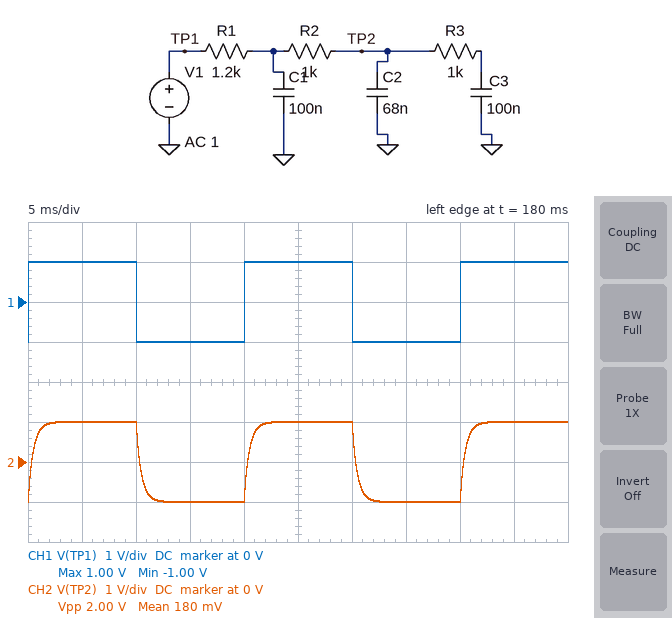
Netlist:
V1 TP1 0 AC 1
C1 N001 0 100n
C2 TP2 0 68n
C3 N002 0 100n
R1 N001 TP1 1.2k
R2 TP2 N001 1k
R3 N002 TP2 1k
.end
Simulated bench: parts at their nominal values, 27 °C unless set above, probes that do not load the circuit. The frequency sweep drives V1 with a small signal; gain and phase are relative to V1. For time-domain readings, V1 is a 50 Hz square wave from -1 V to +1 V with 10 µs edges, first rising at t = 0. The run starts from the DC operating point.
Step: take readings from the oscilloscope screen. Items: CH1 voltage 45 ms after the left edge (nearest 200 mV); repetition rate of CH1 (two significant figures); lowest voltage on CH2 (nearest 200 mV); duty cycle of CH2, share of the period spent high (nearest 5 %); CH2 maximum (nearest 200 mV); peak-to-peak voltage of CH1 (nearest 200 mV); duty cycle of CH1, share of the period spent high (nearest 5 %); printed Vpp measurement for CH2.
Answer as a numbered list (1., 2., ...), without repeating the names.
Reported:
1. 1.0 V
2. 50 Hz
3. -1.0 V
4. 50 %
5. 1.0 V
6. 2.0 V
7. 50 %
8. 2.00 V
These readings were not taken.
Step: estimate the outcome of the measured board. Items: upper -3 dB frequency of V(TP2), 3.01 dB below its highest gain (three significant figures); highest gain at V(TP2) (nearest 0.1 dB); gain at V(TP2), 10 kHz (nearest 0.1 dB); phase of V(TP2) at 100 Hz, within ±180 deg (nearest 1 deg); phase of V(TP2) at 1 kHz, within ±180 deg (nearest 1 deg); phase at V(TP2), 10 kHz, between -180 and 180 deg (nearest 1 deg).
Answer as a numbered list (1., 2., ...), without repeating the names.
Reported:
1. 326 Hz
2. 0 dB
3. -31.8 dB
4. -17 deg
5. -72 deg
6. -141 deg
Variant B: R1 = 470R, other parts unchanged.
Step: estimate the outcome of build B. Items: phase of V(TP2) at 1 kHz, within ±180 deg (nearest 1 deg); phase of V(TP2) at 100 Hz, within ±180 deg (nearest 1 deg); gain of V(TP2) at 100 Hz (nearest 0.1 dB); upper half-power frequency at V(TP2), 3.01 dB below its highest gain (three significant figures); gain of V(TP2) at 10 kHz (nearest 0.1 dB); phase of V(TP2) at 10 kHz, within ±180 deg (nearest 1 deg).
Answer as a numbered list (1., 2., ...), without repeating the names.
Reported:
1. -55 deg
2. -10 deg
3. -0.2 dB
4. 522 Hz
5. -24.2 dB
6. -131 deg
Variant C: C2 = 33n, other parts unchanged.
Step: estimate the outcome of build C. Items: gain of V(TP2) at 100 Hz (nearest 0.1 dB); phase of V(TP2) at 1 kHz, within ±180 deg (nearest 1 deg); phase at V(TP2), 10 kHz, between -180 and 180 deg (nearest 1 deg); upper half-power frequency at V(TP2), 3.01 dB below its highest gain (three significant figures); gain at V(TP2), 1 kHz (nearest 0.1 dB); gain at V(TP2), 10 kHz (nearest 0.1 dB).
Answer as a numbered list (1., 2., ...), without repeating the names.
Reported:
1. -0.3 dB
2. -65 deg
3. -125 deg
4. 378 Hz
5. -8.5 dB
6. -27.6 dB
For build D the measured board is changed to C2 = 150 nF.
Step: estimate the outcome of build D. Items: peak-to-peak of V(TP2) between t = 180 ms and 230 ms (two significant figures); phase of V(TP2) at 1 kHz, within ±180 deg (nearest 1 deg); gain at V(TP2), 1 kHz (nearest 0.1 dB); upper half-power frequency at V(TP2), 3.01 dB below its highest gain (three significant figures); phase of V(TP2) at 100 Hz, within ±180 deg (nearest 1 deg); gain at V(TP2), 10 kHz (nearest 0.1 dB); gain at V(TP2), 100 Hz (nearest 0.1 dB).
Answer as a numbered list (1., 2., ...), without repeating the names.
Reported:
1. 2.0 V
2. -82 deg
3. -12.2 dB
4. 243 Hz
5. -23 deg
6. -37.8 dB
7. -0.7 dB
